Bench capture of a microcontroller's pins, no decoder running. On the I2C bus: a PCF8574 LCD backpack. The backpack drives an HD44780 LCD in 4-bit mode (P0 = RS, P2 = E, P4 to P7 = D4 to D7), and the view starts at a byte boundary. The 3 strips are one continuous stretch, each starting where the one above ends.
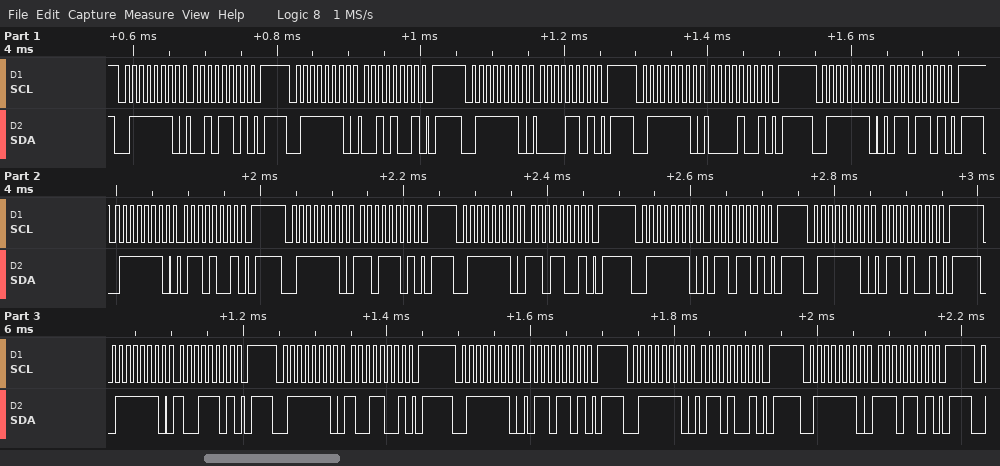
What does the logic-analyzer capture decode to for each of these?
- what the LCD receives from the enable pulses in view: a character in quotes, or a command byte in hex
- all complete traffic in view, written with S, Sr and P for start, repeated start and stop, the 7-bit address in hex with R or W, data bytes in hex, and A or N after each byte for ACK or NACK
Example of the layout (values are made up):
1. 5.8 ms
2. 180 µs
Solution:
1. ' ' 'm' 'i'
2. S 3FW A 2D A P S 3FW A 29 A P S 3FW A 0D A P S 3FW A 09 A P S 3FW A 6D A P S 3FW A 69 A P S 3FW A DD A P S 3FW A D9 A P S 3FW A 6D A P S 3FW A 69 A P S 3FW A 9D A P S 3FW A 99 A P S 3FW A 6D A P S 3FW A 69 A P S 3FW A ED A P
